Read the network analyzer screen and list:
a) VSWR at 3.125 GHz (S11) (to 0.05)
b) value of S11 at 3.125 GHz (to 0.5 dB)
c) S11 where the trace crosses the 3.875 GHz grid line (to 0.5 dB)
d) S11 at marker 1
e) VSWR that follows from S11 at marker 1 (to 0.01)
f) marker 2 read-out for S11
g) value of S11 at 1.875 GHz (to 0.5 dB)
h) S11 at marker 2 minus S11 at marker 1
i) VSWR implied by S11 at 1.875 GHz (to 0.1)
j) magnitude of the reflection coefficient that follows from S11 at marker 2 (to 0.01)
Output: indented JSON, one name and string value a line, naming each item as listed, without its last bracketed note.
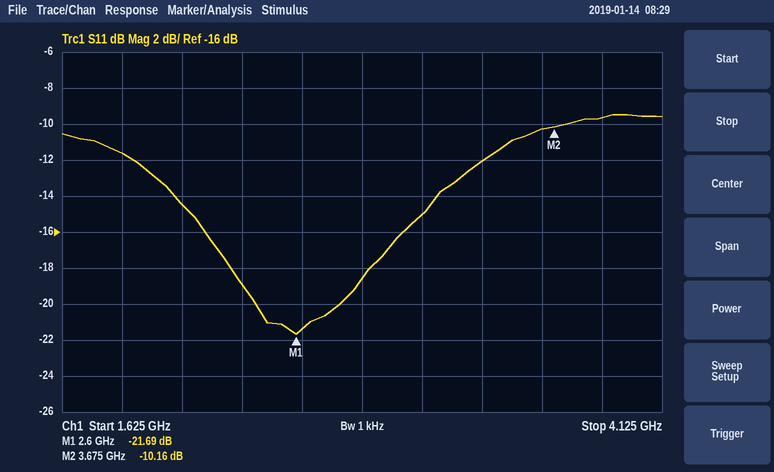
{
  "VSWR at 3.125 GHz (S11)": "1.45",
  "value of S11 at 3.125 GHz": "-15.0 dB",
  "S11 where the trace crosses the 3.875 GHz grid line": "-9.5 dB",
  "S11 at marker 1": "-21.69 dB",
  "VSWR that follows from S11 at marker 1": "1.18",
  "marker 2 read-out for S11": "-10.16 dB",
  "value of S11 at 1.875 GHz": "-11.5 dB",
  "S11 at marker 2 minus S11 at marker 1": "11.53 dB",
  "VSWR implied by S11 at 1.875 GHz": "1.7",
  "magnitude of the reflection coefficient that follows from S11 at marker 2": "0.31"
}
